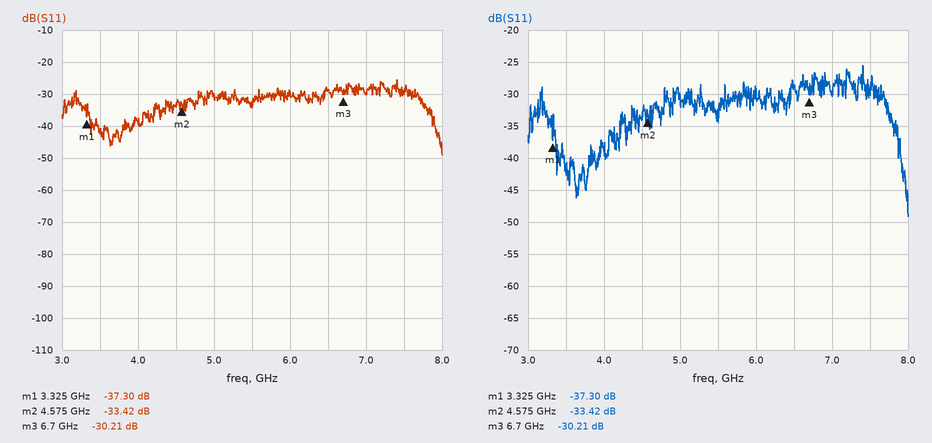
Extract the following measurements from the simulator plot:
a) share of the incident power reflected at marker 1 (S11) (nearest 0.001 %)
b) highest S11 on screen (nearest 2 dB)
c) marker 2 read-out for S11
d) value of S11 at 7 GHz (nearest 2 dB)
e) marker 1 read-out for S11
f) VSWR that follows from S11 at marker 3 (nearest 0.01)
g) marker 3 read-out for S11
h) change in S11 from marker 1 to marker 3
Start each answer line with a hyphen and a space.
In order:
- 0.019 %
- -26 dB
- -33.42 dB
- -30 dB
- -37.30 dB
- 1.06
- -30.21 dB
- 7.09 dB
